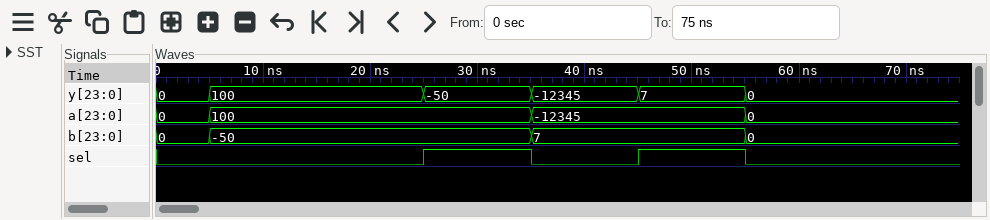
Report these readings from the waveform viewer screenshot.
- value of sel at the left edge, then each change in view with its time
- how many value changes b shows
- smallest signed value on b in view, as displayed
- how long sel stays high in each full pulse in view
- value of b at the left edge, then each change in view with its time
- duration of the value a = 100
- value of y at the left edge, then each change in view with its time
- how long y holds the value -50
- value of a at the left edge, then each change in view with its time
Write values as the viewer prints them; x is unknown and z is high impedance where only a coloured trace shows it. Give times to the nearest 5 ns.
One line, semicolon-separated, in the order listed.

0, 1 at 25 ns, 0 at 35 ns, 1 at 45 ns, 0 at 55 ns; 3; -50; 10 ns, 10 ns; 0, -50 at 5 ns, 7 at 35 ns, 0 at 55 ns; 30 ns; 0, 100 at 5 ns, -50 at 25 ns, -12345 at 35 ns, 7 at 45 ns, 0 at 55 ns; 10 ns; 0, 100 at 5 ns, -12345 at 35 ns, 0 at 55 ns
